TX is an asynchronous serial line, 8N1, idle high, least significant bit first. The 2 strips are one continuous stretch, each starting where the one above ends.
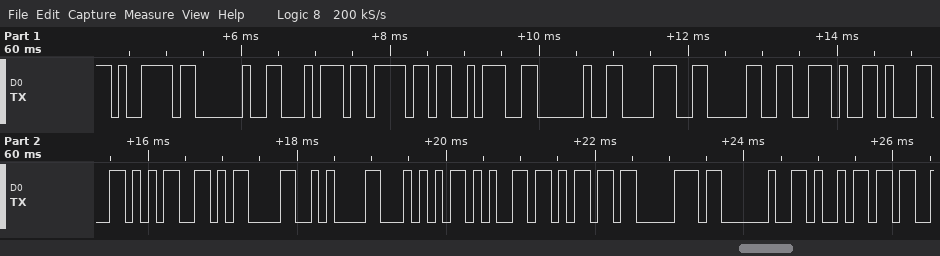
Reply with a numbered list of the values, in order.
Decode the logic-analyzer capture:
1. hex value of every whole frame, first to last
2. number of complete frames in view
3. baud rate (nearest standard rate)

1. 79 20 74 6F 3A 20 38 30 2E 31 35 0D 0A 54 65 6D 70 20 69
2. 19
3. 9600 baud
